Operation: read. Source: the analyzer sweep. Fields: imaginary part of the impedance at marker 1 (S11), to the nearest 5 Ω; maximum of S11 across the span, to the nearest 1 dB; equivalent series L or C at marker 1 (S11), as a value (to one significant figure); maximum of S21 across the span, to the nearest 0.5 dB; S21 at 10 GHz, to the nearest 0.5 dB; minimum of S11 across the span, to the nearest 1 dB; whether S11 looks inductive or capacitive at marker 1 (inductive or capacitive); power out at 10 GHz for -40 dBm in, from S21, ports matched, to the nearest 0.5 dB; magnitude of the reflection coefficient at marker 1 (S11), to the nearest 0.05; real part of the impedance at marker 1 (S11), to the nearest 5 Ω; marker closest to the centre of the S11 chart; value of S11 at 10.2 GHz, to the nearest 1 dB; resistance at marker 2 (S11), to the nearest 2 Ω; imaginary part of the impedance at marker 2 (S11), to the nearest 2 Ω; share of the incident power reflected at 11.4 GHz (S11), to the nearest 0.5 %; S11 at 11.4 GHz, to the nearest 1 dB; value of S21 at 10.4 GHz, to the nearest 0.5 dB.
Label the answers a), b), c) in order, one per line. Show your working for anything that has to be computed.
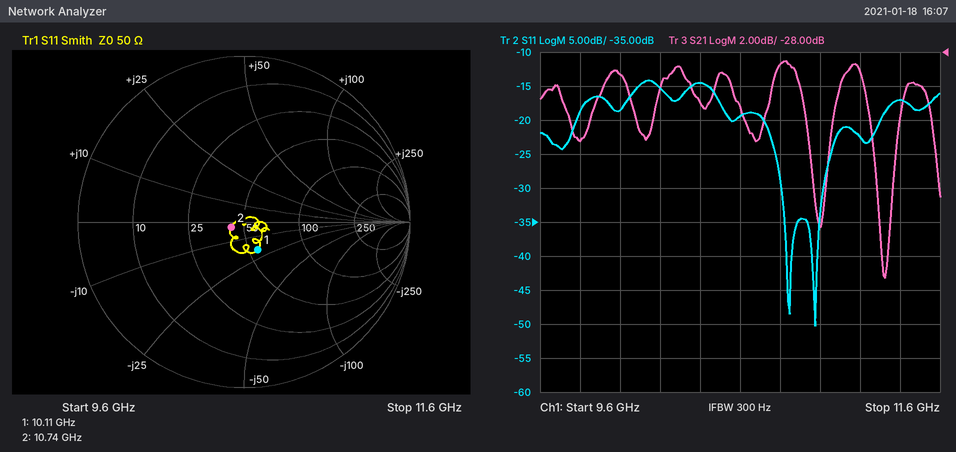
a) -20 Ω
b) -14 dB
c) C = 1/(2π × 10.11 GHz × 20 Ω) ≈ 787 fF, so 800 fF to one significant figure
d) -28.5 dB
e) -29.5 dB
f) -50 dB
g) capacitive
h) -40 dBm + (-29.5 dB) = -69.5 dBm
i) 0.20
j) 55 Ω
k) marker 2
l) -15 dB
m) 42 Ω
n) -2 Ω
o) 10^(-17/10) ≈ 2.0 %
p) -17 dB
q) -31.0 dB
